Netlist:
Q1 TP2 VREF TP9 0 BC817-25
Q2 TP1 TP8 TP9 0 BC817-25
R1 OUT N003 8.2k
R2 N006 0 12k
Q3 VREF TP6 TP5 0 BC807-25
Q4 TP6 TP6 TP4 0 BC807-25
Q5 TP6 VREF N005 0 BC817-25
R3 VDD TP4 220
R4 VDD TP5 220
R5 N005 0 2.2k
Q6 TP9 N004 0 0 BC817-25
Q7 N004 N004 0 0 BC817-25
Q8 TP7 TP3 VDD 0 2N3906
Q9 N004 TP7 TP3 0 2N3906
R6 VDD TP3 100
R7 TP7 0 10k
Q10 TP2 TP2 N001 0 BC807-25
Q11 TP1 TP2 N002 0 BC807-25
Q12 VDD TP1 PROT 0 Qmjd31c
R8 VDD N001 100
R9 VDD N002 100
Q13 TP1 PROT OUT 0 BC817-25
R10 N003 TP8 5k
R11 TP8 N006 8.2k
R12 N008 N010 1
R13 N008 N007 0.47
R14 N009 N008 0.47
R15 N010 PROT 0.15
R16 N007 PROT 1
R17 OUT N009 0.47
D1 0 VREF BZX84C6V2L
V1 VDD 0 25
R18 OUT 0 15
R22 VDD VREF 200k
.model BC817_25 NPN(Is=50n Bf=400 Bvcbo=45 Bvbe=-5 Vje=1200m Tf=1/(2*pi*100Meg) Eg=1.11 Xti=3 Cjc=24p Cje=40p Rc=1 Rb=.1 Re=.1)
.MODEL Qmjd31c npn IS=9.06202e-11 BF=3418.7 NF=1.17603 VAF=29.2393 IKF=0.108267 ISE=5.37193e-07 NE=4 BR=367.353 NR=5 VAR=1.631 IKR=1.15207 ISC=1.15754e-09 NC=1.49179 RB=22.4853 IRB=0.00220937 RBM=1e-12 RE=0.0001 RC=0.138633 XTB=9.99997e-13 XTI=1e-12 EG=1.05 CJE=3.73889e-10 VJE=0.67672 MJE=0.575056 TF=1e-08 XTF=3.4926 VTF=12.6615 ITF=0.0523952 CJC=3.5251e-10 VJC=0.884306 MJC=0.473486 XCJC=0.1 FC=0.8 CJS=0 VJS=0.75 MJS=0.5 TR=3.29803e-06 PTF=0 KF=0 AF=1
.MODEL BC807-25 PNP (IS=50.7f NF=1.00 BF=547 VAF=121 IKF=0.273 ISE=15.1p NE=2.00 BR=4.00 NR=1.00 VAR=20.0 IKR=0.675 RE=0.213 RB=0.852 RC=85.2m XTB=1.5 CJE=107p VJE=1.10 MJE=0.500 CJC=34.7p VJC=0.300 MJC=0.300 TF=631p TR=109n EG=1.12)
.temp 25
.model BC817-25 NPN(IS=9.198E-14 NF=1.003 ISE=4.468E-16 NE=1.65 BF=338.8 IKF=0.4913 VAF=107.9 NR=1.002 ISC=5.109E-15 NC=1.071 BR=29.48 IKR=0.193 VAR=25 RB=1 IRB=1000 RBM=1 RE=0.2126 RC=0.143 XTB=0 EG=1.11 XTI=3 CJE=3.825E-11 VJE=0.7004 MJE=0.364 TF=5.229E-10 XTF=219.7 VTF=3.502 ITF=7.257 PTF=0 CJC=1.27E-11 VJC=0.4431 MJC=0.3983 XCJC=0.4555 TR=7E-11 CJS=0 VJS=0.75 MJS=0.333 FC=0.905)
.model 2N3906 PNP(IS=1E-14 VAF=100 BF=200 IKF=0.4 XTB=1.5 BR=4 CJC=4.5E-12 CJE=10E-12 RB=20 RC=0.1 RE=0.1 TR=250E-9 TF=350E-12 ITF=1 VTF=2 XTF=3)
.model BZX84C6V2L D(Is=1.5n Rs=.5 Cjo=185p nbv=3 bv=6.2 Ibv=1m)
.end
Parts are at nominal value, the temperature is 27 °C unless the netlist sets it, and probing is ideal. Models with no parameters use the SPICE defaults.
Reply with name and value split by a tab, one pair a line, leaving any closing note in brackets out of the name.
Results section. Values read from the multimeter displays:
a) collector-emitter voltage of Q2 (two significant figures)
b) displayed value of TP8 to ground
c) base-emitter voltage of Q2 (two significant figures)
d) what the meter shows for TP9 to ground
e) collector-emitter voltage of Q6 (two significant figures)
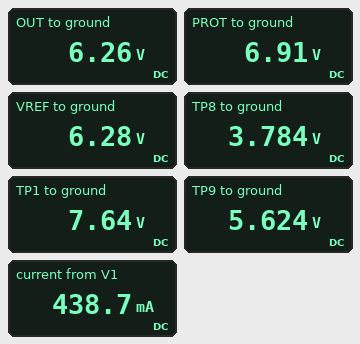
collector-emitter voltage of Q2	2.0 V
displayed value of TP8 to ground	3.784 V
base-emitter voltage of Q2	-1.8 V
what the meter shows for TP9 to ground	5.624 V
collector-emitter voltage of Q6	5.6 V
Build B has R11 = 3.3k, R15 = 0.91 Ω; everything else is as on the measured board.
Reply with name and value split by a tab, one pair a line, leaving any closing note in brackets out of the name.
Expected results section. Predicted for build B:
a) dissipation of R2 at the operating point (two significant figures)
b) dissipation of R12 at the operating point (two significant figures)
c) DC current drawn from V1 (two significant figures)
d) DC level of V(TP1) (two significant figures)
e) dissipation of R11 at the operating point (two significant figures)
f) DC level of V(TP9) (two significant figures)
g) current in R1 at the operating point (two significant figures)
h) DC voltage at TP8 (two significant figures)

dissipation of R2 at the operating point	470 µW
dissipation of R12 at the operating point	26 mW
DC current drawn from V1	400 mA
DC level of V(TP1)	7.0 V
dissipation of R11 at the operating point	130 µW
DC level of V(TP9)	5.6 V
current in R1 at the operating point	200 µA
DC voltage at TP8	3.0 V
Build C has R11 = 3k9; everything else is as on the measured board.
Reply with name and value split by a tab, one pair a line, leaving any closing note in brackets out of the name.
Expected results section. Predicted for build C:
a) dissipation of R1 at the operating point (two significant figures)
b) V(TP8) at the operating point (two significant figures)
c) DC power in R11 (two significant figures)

dissipation of R1 at the operating point	380 µW
V(TP8) at the operating point	3.4 V
DC power in R11	180 µW
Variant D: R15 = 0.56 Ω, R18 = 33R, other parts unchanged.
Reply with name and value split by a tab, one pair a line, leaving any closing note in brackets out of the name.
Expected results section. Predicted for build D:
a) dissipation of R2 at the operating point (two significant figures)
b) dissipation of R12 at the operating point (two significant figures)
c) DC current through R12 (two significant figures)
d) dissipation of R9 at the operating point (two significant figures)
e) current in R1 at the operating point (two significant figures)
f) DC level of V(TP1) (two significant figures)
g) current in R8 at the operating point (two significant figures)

dissipation of R2 at the operating point	1.2 mW
dissipation of R12 at the operating point	24 mW
DC current through R12	150 mA
dissipation of R9 at the operating point	1.6 mW
current in R1 at the operating point	320 µA
DC level of V(TP1)	12 V
current in R8 at the operating point	4.0 mA
